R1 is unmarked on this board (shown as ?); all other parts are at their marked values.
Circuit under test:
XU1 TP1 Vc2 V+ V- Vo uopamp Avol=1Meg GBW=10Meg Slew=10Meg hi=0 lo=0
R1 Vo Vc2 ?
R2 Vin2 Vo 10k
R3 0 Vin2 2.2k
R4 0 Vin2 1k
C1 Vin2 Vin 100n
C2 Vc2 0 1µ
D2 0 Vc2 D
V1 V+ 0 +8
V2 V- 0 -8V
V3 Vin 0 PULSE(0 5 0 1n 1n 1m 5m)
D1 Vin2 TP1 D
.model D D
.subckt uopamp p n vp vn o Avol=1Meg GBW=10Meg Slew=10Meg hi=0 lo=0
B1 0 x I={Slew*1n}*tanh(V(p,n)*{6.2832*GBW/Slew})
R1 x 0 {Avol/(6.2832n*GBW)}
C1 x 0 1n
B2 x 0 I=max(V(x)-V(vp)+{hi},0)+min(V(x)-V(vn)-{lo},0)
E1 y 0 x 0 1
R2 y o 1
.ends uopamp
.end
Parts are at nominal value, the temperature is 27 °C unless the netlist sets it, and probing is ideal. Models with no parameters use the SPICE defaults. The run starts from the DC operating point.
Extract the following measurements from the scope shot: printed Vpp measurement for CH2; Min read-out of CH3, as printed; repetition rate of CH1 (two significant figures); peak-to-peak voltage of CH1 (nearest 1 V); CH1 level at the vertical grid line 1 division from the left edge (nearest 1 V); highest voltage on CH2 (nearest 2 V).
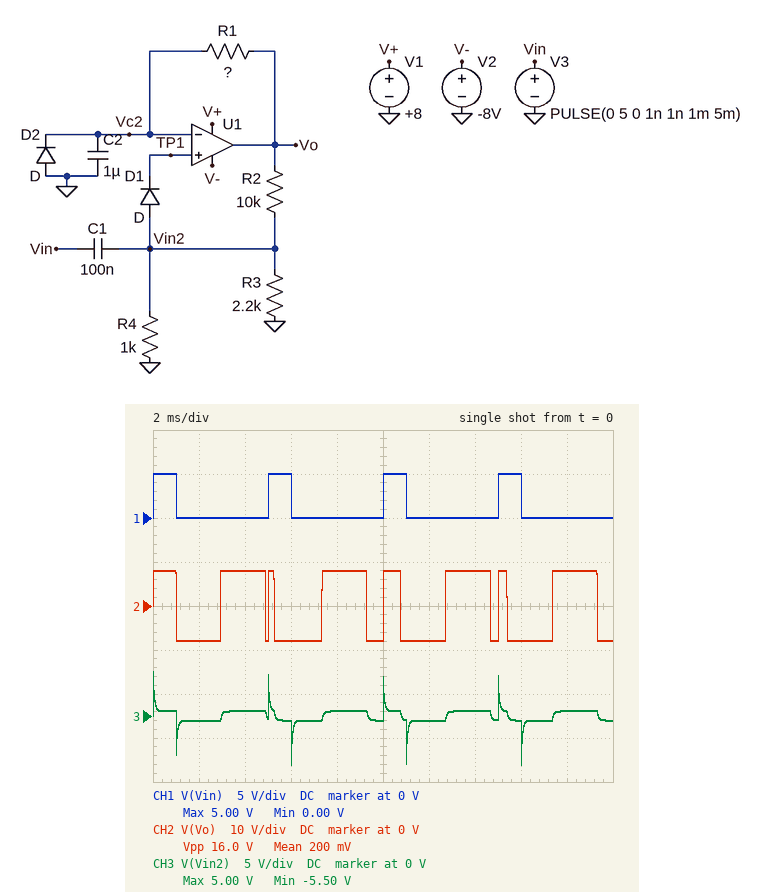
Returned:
16.0 V
-5.50 V
200 Hz
5 V
0 V
8 V
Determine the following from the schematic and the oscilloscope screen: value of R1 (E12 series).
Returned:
15 kΩ
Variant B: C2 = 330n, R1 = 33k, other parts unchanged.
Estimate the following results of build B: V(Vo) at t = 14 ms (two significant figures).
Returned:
-8.0 V
